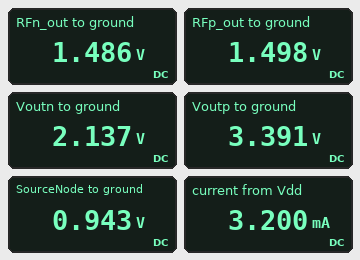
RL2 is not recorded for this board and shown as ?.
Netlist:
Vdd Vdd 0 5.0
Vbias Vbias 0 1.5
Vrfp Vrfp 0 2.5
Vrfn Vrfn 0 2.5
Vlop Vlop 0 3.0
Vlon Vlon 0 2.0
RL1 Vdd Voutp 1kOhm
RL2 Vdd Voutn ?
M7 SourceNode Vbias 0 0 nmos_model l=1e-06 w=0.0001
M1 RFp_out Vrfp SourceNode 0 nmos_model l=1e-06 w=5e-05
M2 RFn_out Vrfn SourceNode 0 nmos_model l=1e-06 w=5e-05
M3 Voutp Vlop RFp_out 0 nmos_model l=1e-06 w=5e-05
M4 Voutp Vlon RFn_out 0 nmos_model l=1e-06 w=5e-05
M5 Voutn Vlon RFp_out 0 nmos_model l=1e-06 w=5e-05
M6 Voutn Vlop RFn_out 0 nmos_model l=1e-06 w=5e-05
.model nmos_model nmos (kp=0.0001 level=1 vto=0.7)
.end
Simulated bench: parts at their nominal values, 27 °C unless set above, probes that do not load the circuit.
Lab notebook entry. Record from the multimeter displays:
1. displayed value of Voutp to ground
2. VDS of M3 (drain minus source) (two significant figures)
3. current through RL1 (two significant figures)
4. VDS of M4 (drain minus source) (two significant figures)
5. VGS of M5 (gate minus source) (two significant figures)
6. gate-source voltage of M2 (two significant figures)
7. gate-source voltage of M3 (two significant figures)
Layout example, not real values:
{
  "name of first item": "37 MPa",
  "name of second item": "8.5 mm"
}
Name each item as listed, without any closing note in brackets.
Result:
{
  "displayed value of Voutp to ground": "3.391 V",
  "VDS of M3 (drain minus source)": "1.9 V",
  "current through RL1": "1.6 mA",
  "VDS of M4 (drain minus source)": "1.9 V",
  "VGS of M5 (gate minus source)": "500 mV",
  "gate-source voltage of M2": "1.6 V",
  "gate-source voltage of M3": "1.5 V"
}
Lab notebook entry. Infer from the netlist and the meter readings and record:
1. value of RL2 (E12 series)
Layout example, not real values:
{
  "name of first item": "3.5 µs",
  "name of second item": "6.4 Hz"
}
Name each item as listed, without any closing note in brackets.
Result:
{
  "value of RL2": "1.8 kΩ"
}
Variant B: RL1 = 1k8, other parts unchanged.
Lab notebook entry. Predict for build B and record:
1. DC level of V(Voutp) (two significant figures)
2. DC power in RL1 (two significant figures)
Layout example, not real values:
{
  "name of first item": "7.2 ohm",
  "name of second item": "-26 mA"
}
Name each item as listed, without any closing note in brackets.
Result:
{
  "DC level of V(Voutp)": "2.1 V",
  "DC power in RL1": "4.6 mW"
}
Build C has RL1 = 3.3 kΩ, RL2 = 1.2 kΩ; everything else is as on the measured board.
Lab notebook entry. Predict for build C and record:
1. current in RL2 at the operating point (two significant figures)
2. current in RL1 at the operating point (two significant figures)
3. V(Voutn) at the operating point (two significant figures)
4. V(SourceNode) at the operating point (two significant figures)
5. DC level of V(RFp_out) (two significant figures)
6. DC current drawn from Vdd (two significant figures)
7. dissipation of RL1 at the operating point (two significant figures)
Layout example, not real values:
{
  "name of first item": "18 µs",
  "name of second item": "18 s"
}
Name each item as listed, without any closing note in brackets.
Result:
{
  "current in RL2 at the operating point": "2.1 mA",
  "current in RL1 at the operating point": "1.1 mA",
  "V(Voutn) at the operating point": "2.5 V",
  "V(SourceNode) at the operating point": "820 mV",
  "DC level of V(RFp_out)": "1.1 V",
  "DC current drawn from Vdd": "3.2 mA",
  "dissipation of RL1 at the operating point": "4.1 mW"
}
